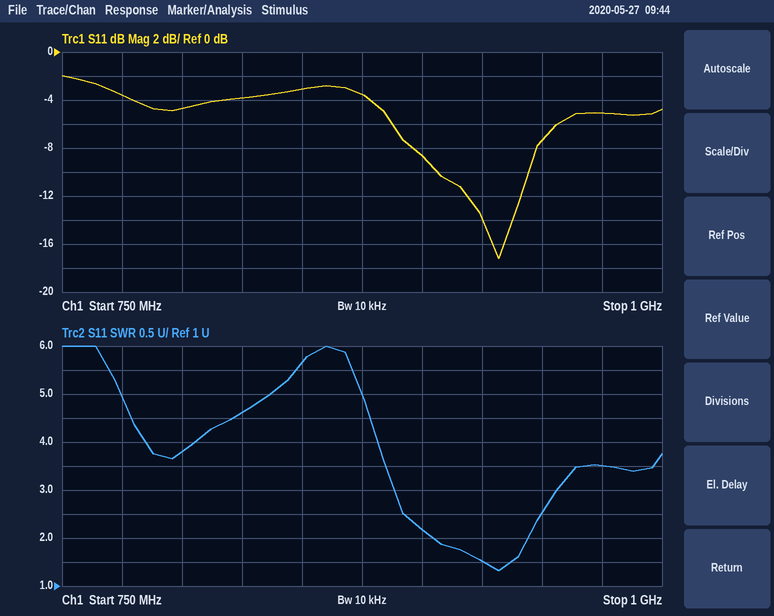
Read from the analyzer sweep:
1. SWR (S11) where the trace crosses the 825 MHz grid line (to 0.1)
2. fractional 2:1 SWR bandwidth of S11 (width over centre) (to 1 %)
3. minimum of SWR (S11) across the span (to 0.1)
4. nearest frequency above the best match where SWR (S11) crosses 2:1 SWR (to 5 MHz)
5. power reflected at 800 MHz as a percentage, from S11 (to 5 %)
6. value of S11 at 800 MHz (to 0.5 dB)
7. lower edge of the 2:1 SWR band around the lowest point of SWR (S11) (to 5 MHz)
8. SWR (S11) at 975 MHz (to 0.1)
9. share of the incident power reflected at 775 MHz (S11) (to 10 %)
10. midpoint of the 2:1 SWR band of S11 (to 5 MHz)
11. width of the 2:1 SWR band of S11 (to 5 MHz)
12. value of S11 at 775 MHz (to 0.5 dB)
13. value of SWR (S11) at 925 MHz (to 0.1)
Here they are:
4.6
4 %
1.3
945 MHz
35 %
-4.5 dB
905 MHz
3.5
40 %
925 MHz
40 MHz
-3.5 dB
1.5
